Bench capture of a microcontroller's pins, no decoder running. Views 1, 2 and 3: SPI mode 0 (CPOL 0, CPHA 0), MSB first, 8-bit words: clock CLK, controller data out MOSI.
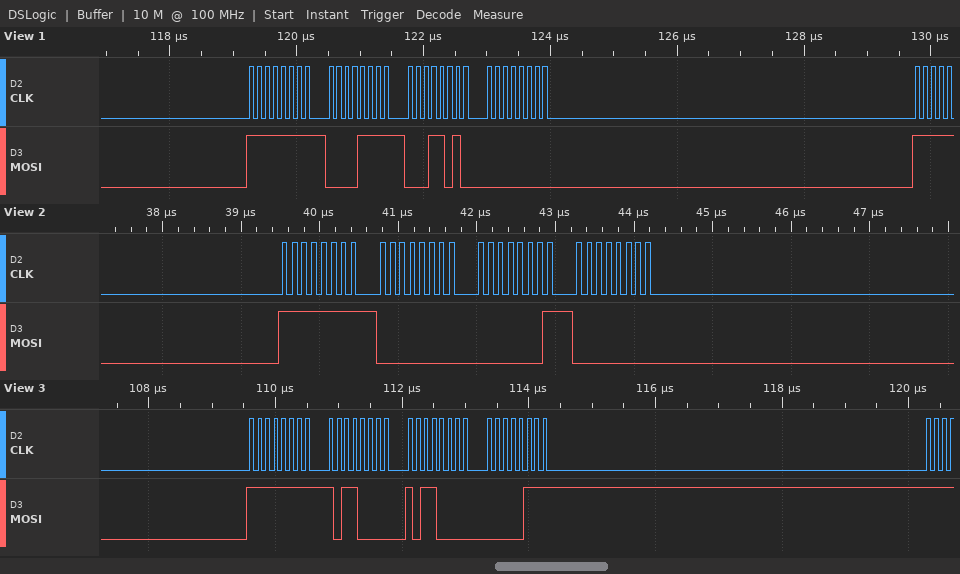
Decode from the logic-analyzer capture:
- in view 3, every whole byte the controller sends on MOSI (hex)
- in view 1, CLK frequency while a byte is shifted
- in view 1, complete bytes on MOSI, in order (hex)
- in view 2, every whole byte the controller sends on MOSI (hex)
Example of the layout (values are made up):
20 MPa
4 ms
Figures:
0xFF 0xB0 0xB0 0x07
8 MHz
FF 0F 1A 00
0xFF 0x00 0x01 0x00
